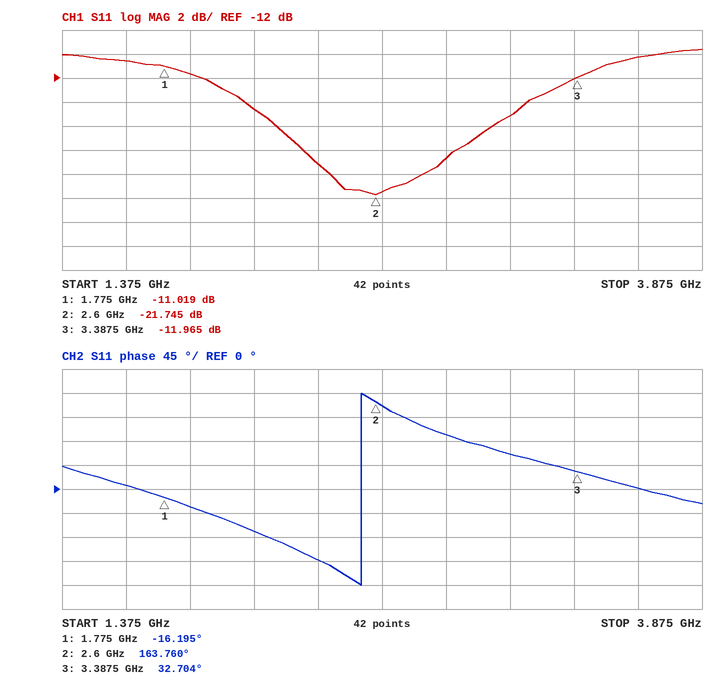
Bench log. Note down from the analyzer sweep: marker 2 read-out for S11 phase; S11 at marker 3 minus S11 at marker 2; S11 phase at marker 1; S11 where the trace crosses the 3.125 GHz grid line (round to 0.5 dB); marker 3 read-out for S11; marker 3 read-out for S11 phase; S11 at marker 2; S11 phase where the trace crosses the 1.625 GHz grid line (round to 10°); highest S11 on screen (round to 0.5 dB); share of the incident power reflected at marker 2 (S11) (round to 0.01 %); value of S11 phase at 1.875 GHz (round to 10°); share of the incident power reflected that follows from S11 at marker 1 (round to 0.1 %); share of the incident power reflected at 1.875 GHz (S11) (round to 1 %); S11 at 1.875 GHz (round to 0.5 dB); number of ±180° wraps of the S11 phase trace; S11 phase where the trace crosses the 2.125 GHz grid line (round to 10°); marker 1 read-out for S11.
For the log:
163.760°
9.780 dB
-16.195°
-15.0 dB
-11.965 dB
32.704°
-21.745 dB
10°
-9.5 dB
0.67 %
-30°
7.9 %
7 %
-11.5 dB
1
-80°
-11.019 dB
